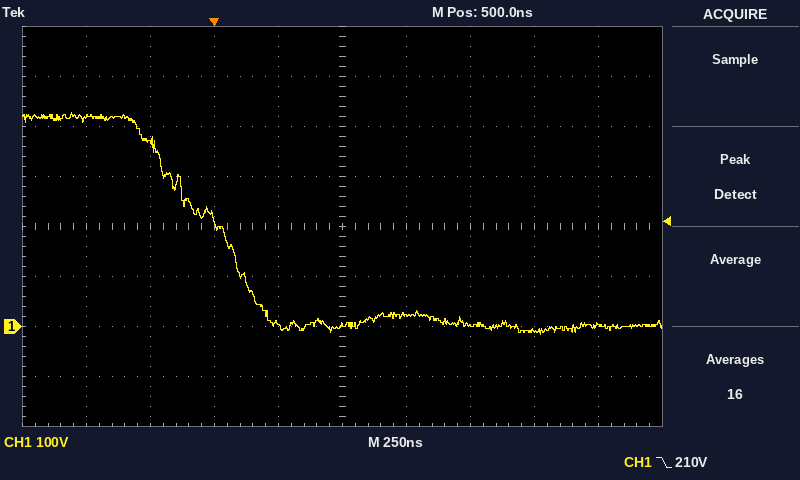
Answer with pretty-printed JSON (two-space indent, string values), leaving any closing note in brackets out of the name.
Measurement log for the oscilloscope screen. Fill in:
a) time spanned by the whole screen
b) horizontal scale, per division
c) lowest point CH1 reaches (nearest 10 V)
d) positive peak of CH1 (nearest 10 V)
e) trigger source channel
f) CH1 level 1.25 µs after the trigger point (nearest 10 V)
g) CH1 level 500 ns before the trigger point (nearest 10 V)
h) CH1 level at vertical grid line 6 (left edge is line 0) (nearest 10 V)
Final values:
{
  "time spanned by the whole screen": "2.5 µs",
  "horizontal scale, per division": "250 ns",
  "lowest point CH1 reaches": "-20 V",
  "positive peak of CH1": "430 V",
  "trigger source channel": "CH1",
  "CH1 level 1.25 µs after the trigger point": "-10 V",
  "CH1 level 500 ns before the trigger point": "420 V",
  "CH1 level at vertical grid line 6 (left edge is line 0)": "20 V"
}
